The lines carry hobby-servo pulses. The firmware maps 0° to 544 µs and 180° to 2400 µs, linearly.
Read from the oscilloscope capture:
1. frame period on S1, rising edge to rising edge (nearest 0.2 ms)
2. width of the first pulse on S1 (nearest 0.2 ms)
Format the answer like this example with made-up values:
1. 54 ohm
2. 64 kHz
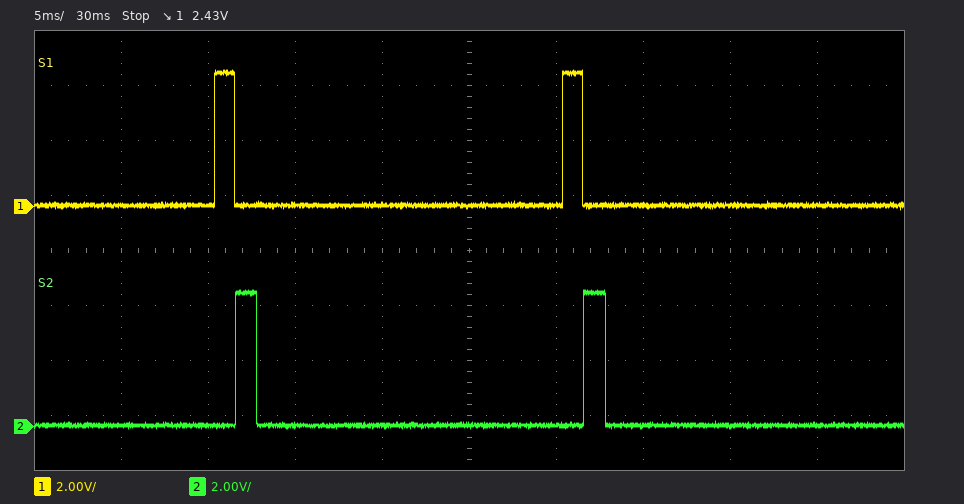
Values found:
1. 20.0 ms
2. 1.2 ms
